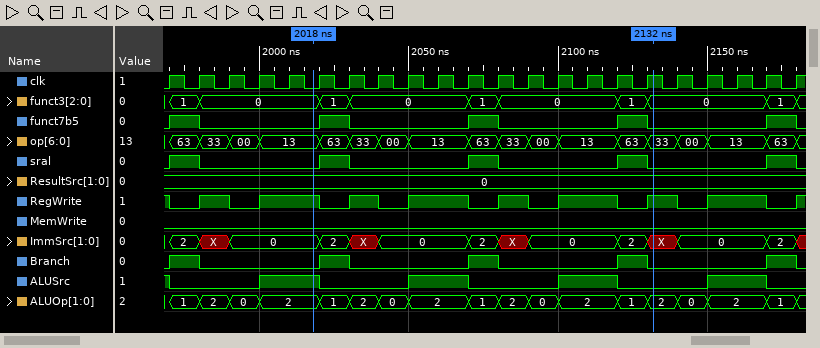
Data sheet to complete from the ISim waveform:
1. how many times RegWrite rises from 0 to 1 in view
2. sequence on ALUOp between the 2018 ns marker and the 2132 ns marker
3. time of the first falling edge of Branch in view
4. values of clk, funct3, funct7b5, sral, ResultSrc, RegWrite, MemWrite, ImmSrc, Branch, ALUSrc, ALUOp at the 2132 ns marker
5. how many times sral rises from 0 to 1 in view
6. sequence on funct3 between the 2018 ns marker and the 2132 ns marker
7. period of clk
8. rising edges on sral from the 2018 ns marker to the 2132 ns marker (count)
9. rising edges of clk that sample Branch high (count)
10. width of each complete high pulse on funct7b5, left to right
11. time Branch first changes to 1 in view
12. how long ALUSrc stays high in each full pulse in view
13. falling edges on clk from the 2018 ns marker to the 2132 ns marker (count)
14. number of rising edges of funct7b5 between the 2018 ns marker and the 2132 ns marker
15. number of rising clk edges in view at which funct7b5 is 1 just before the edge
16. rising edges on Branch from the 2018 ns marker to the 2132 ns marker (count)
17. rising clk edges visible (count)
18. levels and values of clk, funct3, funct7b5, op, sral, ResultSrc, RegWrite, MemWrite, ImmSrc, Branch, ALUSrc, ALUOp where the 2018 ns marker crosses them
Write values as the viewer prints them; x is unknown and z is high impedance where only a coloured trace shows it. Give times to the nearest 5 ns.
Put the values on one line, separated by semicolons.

9; 2, 1, 2, 0, 2, 1, 2, 0, 2, 1, 2; 1980 ns; clk=1, funct3=0, funct7b5=0, sral=0, ResultSrc=0, RegWrite=1, MemWrite=0, ImmSrc=X, Branch=0, ALUSrc=0, ALUOp=2; 5; 0, 1, 0, 1, 0, 1, 0; 10 ns; 3; 5; 10 ns, 10 ns, 10 ns, 10 ns, 10 ns; 1970 ns; 20 ns, 20 ns, 20 ns, 20 ns; 11; 3; 5; 3; 22; clk=0, funct3=0, funct7b5=0, op=13, sral=0, ResultSrc=0, RegWrite=1, MemWrite=0, ImmSrc=0, Branch=0, ALUSrc=1, ALUOp=2
